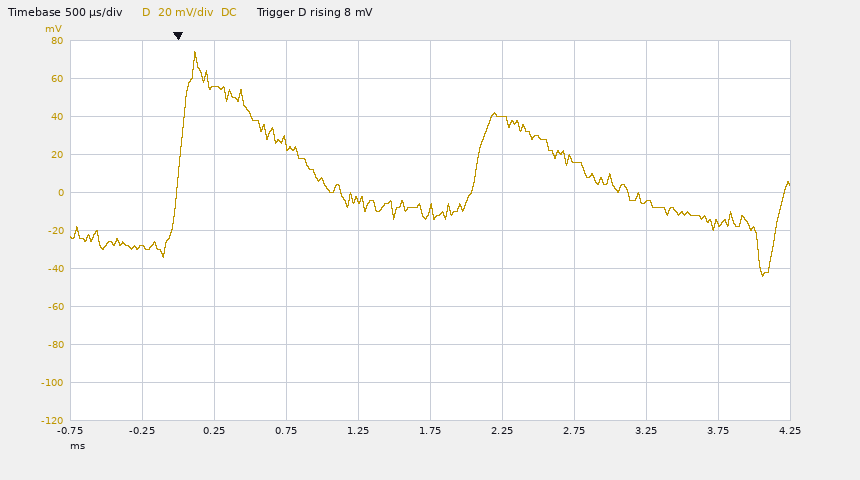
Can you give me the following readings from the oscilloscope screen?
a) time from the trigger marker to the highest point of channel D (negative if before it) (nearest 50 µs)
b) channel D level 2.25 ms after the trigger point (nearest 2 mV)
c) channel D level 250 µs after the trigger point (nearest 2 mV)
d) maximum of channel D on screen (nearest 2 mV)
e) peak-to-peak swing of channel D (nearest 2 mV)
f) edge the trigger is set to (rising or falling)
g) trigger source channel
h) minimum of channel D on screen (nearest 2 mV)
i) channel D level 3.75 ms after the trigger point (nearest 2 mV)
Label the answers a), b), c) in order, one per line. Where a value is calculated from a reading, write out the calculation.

a) +100 µs
b) 40 mV
c) 56 mV
d) 74 mV
e) 74 mV − (-44 mV) = 118 mV
f) rising
g) channel D
h) -44 mV
i) -16 mV
